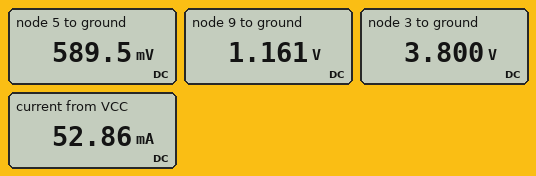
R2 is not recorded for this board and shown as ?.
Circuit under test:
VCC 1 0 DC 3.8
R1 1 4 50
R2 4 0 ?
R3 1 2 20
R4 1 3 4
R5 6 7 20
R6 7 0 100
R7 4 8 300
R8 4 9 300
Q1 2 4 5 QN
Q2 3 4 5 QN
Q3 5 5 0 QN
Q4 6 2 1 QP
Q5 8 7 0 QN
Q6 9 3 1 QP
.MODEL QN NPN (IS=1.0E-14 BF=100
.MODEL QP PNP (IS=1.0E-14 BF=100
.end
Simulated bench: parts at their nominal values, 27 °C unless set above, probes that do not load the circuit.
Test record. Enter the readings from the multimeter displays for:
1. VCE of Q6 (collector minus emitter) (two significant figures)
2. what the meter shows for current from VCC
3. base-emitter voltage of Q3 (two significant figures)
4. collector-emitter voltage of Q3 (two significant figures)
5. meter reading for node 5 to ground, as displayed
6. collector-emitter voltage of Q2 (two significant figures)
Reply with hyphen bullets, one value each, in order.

- -2.6 V
- 52.86 mA
- 590 mV
- 590 mV
- 589.5 mV
- 3.2 V
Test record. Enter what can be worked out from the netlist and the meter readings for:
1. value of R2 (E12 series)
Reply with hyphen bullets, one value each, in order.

- 22 Ω
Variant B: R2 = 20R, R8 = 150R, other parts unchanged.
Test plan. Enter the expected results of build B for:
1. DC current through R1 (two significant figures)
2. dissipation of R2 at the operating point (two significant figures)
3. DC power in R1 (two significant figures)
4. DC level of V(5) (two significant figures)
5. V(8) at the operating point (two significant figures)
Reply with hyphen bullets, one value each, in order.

- 54 mA
- 59 mW
- 150 mW
- 550 mV
- 1.1 V
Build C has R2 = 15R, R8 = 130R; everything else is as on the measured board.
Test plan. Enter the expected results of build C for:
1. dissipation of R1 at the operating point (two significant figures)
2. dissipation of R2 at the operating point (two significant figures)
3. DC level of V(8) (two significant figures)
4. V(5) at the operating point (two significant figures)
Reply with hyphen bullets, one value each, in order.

- 170 mW
- 51 mW
- 880 mV
- 450 mV
